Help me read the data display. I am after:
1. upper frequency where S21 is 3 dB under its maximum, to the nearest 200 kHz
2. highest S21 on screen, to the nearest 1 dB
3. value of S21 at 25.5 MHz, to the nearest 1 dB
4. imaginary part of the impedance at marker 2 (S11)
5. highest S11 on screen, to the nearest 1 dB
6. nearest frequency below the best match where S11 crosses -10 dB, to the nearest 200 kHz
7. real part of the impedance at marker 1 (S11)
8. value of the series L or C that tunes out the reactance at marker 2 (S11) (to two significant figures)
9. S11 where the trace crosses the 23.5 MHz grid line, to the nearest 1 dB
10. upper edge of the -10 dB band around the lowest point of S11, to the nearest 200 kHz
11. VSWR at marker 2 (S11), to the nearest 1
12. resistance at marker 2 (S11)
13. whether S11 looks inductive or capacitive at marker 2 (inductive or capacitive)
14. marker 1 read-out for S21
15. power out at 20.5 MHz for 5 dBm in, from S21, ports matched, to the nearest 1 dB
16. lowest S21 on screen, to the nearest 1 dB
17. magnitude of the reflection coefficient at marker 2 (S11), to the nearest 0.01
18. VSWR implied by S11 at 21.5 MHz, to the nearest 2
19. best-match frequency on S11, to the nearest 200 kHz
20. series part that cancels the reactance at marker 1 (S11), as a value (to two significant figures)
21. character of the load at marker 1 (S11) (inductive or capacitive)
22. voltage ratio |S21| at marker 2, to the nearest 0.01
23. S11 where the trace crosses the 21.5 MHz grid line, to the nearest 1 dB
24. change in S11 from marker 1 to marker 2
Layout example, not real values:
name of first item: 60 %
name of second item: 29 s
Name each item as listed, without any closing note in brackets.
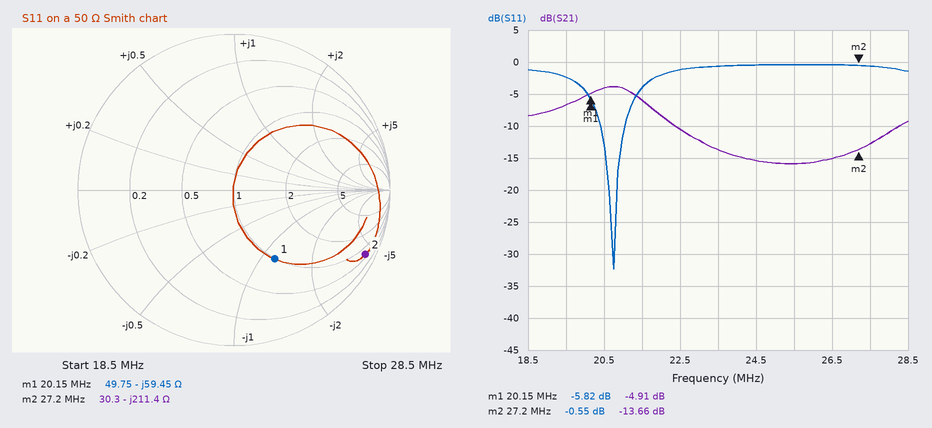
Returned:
upper frequency where S21 is 3 dB under its maximum, to the nearest 200 kHz: 21.6 MHz
highest S21 on screen, to the nearest 1 dB: -4 dB
value of S21 at 25.5 MHz, to the nearest 1 dB: -16 dB
imaginary part of the impedance at marker 2: -211.4 Ω
highest S11 on screen, to the nearest 1 dB: 0 dB
nearest frequency below the best match where S11 crosses -10 dB, to the nearest 200 kHz: 20.4 MHz
real part of the impedance at marker 1: 49.75 Ω
value of the series L or C that tunes out the reactance at marker 2 (S11): 1.2 µH
S11 where the trace crosses the 23.5 MHz grid line, to the nearest 1 dB: -1 dB
upper edge of the -10 dB band around the lowest point of S11, to the nearest 200 kHz: 21.0 MHz
VSWR at marker 2 (S11), to the nearest 1: 32
resistance at marker 2: 30.3 Ω
whether S11 looks inductive or capacitive at marker 2: capacitive
marker 1 read-out for S21: -4.91 dB
power out at 20.5 MHz for 5 dBm in, from S21, ports matched, to the nearest 1 dB: 1 dBm
lowest S21 on screen, to the nearest 1 dB: -16 dB
magnitude of the reflection coefficient at marker 2 (S11), to the nearest 0.01: 0.94
VSWR implied by S11 at 21.5 MHz, to the nearest 2: 4
best-match frequency on S11, to the nearest 200 kHz: 20.8 MHz
series part that cancels the reactance at marker 1 (S11), as a value: 470 nH
character of the load at marker 1 (S11): capacitive
voltage ratio |S21| at marker 2, to the nearest 0.01: 0.21
S11 where the trace crosses the 21.5 MHz grid line, to the nearest 1 dB: -4 dB
change in S11 from marker 1 to marker 2: 5.27 dB
